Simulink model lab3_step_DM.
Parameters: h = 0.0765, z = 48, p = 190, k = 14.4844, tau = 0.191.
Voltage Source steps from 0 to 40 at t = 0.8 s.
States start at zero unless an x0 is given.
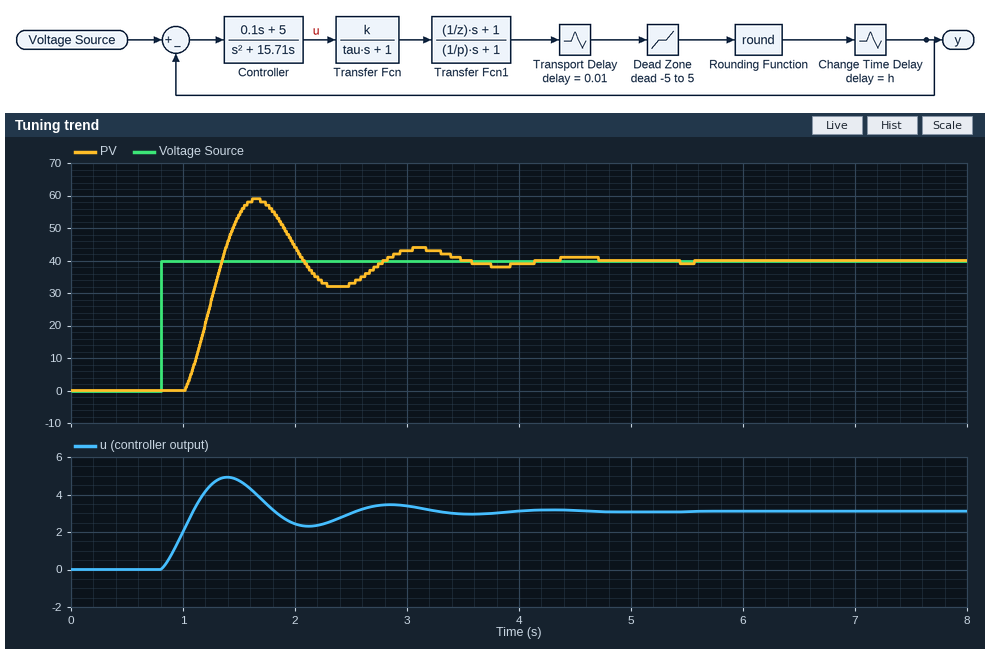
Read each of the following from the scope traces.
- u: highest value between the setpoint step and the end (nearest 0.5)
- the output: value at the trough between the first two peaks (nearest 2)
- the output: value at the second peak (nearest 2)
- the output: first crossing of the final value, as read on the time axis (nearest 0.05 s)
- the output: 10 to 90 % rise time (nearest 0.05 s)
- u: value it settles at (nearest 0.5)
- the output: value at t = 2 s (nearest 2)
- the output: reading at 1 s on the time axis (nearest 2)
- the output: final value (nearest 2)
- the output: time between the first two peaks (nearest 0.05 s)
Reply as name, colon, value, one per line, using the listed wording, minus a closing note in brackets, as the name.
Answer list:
u: highest value between the setpoint step and the end: 5.0
the output: value at the trough between the first two peaks: 32
the output: value at the second peak: 44
the output: first crossing of the final value, as read on the time axis: 1.35 s
the output: 10 to 90 % rise time: 0.25 s
u: value it settles at: 3.0
the output: value at t = 2 s: 44
the output: reading at 1 s on the time axis: 0
the output: final value: 40
the output: time between the first two peaks: 1.45 s
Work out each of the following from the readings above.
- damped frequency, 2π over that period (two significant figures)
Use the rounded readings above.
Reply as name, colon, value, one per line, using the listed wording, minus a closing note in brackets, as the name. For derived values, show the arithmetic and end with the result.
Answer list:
damped frequency, 2π over that period: 2π / 1.45 = 4.3 rad/s
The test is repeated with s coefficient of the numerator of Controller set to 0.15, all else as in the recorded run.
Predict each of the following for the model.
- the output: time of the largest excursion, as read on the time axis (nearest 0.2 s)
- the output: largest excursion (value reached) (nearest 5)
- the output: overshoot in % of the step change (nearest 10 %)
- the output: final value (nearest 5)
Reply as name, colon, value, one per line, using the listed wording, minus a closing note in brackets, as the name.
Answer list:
the output: time of the largest excursion, as read on the time axis: 1.6 s
the output: largest excursion (value reached): 55
the output: overshoot in % of the step change: 40 %
the output: final value: 40
